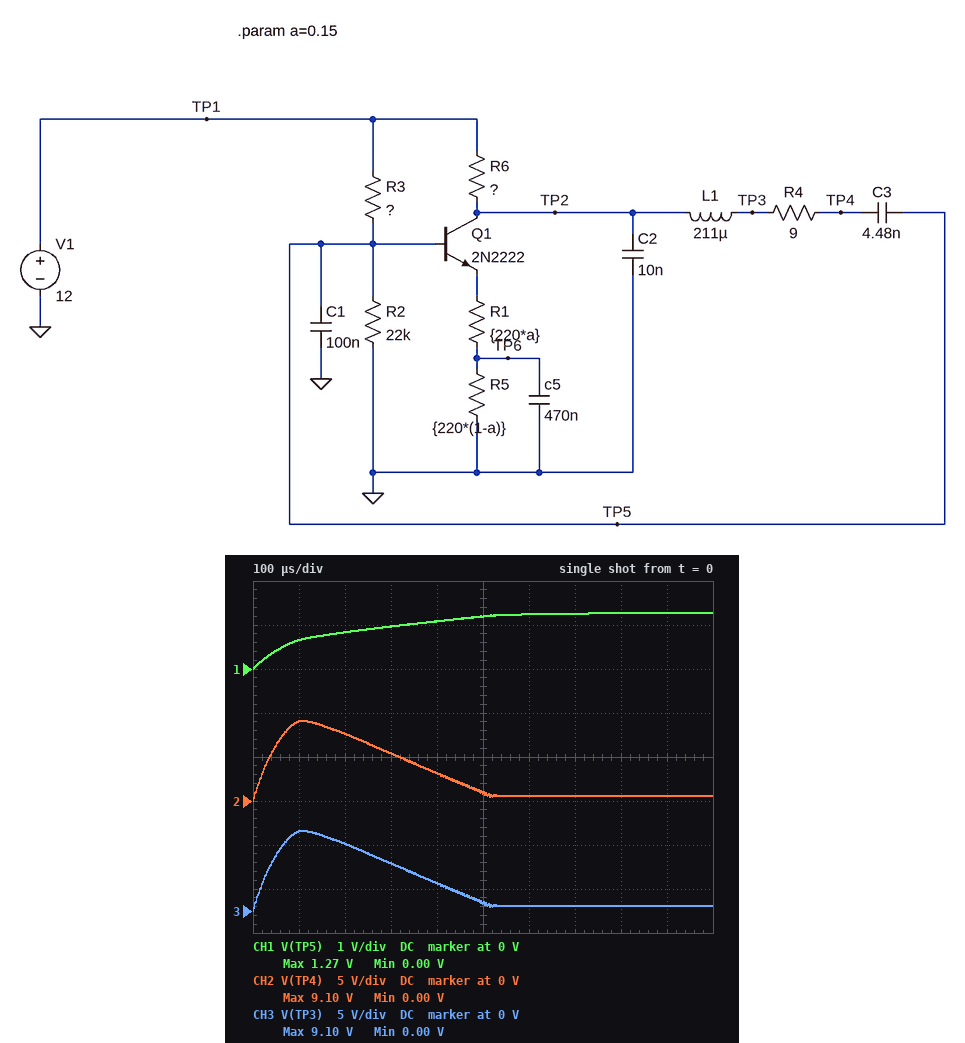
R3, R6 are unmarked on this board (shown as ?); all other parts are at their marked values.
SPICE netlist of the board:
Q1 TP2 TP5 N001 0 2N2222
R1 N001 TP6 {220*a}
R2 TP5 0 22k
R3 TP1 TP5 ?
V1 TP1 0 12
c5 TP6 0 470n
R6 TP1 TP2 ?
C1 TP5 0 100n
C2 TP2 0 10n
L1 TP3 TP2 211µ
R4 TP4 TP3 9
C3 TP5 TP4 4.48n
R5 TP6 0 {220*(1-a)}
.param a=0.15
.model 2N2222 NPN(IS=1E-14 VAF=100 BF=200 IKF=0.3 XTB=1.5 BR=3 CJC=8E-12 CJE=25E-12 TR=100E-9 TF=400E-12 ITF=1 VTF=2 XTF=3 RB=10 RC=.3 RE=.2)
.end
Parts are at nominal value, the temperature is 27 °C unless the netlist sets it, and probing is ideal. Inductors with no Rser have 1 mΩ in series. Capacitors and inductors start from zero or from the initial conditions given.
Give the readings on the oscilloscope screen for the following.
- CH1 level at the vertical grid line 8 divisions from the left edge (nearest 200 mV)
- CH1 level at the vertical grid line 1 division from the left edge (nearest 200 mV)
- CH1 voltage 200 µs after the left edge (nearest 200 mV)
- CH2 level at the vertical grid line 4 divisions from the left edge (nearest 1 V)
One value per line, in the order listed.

1.2 V
600 mV
800 mV
3 V
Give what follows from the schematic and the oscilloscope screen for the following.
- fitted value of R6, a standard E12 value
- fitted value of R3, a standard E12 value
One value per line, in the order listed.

4.7 kΩ
39 kΩ
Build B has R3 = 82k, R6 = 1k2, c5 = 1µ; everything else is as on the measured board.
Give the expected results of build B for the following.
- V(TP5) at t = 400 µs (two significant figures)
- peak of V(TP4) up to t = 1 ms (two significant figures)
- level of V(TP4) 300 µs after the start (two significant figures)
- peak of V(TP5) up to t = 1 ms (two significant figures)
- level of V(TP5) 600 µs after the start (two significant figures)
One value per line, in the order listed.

850 mV
12 V
11 V
1.2 V
990 mV
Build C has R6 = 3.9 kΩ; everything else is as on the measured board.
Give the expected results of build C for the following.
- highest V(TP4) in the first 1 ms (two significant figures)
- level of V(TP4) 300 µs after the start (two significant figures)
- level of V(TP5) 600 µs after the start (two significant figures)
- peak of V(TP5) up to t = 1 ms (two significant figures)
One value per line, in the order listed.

9.6 V
6.0 V
1.3 V
1.4 V
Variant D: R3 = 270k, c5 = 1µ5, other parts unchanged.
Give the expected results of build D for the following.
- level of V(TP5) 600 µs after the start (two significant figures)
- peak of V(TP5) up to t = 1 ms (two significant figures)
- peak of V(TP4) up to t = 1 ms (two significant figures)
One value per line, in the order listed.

610 mV
640 mV
12 V
